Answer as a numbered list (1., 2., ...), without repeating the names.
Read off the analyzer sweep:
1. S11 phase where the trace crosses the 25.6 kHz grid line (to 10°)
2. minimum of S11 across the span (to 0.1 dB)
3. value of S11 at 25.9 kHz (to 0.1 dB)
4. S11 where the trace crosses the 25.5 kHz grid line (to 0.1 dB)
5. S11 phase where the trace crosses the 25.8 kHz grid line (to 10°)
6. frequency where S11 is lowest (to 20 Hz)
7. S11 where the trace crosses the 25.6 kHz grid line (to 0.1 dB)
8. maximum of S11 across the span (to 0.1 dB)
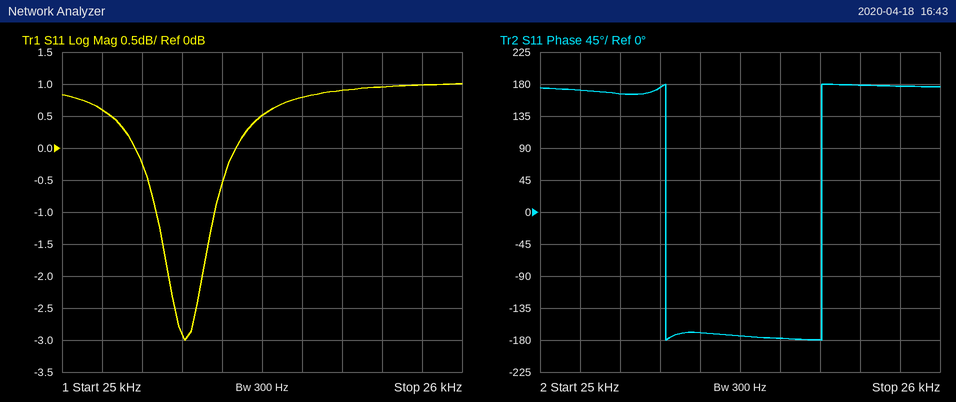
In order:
1. -180°
2. -3.0 dB
3. 1.0 dB
4. 0.5 dB
5. 180°
6. 25.30 kHz
7. 0.8 dB
8. 1.0 dB
